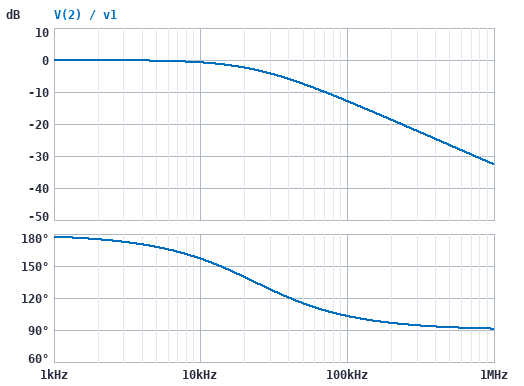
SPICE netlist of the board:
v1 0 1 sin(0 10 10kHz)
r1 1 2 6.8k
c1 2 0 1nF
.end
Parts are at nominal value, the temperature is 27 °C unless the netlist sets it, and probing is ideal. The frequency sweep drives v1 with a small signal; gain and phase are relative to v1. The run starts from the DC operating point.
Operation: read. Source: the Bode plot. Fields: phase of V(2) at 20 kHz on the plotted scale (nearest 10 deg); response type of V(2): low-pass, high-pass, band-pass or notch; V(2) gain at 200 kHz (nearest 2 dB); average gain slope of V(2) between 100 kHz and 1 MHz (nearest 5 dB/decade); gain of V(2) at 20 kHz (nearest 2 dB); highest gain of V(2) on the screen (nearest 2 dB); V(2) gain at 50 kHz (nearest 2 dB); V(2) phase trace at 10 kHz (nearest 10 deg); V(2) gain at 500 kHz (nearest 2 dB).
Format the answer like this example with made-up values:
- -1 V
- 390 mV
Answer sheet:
- 140 deg
- low-pass
- -18 dB
- -20 dB/decade
- -2 dB
- 0 dB
- -8 dB
- 160 deg
- -26 dB
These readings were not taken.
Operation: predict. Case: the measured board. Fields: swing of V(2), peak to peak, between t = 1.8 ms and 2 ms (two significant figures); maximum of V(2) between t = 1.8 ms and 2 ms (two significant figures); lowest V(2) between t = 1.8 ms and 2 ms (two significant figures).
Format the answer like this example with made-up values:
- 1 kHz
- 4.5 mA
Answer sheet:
- 18 V
- 9.2 V
- -9.2 V
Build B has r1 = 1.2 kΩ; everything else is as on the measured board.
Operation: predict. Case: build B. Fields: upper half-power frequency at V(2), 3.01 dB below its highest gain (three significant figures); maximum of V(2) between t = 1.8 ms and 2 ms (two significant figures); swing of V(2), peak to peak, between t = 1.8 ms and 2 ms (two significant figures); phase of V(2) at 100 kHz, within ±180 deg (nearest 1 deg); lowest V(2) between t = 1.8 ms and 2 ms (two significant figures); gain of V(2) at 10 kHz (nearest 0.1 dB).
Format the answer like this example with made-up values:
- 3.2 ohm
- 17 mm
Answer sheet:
- 133 kHz
- 10 V
- 20 V
- 143 deg
- -10 V
- 0 dB
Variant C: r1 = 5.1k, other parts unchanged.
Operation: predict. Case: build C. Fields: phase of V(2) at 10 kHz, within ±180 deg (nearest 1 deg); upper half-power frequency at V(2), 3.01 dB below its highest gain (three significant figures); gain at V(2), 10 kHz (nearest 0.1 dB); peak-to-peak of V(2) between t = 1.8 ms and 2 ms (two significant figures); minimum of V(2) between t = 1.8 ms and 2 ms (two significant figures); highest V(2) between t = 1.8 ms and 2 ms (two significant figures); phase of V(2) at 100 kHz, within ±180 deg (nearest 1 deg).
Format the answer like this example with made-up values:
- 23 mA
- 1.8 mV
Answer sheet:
- 162 deg
- 31.2 kHz
- -0.4 dB
- 19 V
- -9.5 V
- 9.5 V
- 107 deg
